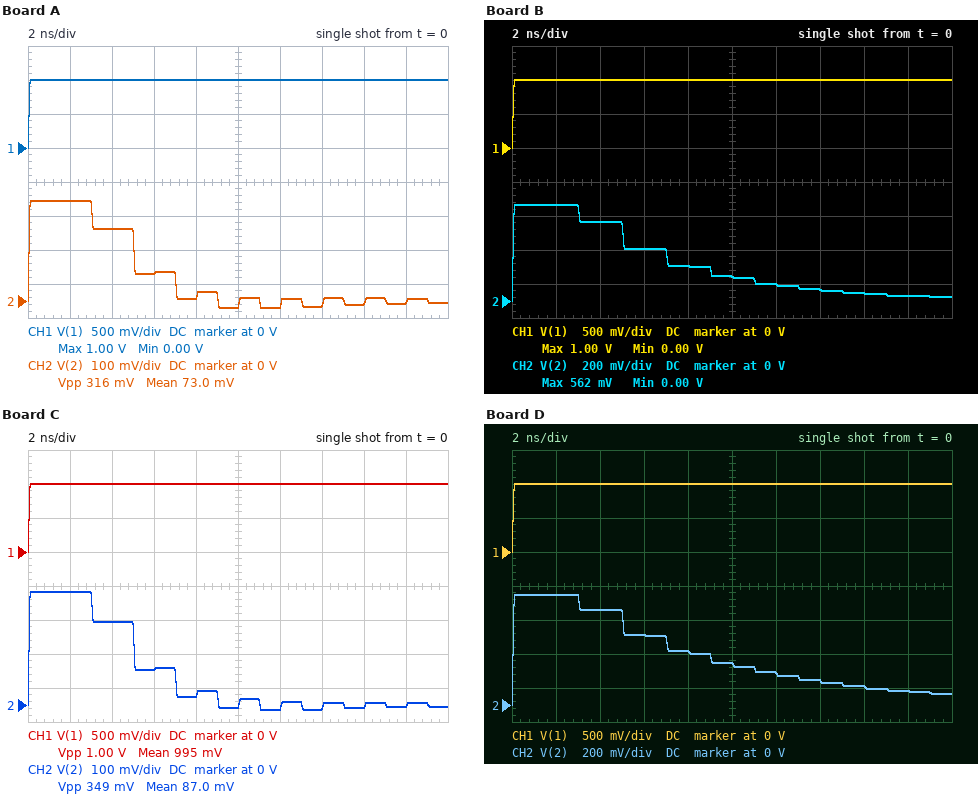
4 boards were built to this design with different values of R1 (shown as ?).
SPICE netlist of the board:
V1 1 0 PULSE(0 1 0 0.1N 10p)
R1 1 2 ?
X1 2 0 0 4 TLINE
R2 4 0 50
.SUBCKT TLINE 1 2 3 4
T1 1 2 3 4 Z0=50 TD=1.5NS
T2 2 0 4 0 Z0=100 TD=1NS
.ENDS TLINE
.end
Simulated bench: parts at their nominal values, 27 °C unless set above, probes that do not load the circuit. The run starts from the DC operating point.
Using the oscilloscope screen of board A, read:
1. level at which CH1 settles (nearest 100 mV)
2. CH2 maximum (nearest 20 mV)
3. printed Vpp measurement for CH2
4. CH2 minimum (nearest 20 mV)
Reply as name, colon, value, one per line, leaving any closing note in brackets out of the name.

level at which CH1 settles: 1.0 V
CH2 maximum: 300 mV
printed Vpp measurement for CH2: 316 mV
CH2 minimum: -20 mV
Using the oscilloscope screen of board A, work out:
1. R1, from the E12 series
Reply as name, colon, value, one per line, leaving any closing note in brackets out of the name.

R1, from the E12 series: 120 Ω
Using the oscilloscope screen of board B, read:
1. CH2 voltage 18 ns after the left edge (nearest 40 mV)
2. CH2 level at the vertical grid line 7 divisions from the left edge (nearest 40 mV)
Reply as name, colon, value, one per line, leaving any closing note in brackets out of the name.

CH2 voltage 18 ns after the left edge: 40 mV
CH2 level at the vertical grid line 7 divisions from the left edge: 80 mV
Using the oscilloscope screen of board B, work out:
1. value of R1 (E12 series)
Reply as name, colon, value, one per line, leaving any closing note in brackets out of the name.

value of R1: 39 Ω
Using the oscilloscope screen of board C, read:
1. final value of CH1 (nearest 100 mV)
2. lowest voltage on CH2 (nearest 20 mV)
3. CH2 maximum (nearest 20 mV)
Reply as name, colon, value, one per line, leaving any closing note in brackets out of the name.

final value of CH1: 1.0 V
lowest voltage on CH2: -20 mV
CH2 maximum: 340 mV
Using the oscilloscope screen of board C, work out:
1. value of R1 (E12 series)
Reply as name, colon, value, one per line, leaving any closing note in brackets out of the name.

value of R1: 100 Ω
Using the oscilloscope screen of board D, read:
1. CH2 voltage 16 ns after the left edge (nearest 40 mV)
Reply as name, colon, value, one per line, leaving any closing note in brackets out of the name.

CH2 voltage 16 ns after the left edge: 120 mV
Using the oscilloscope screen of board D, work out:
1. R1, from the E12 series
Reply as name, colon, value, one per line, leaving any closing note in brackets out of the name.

R1, from the E12 series: 27 Ω
